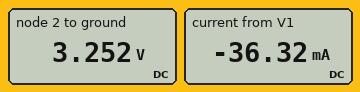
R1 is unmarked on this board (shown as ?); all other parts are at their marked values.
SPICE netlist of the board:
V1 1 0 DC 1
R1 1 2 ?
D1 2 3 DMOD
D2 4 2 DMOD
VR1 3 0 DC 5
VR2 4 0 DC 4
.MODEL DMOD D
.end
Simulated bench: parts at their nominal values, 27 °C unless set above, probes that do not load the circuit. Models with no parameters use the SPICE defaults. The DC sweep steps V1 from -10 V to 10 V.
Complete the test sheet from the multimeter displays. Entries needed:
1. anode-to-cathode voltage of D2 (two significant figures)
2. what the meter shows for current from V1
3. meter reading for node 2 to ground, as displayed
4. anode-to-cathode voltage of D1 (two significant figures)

750 mV
-36.32 mA
3.252 V
-1.7 V
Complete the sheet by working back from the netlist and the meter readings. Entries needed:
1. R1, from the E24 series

62 Ω
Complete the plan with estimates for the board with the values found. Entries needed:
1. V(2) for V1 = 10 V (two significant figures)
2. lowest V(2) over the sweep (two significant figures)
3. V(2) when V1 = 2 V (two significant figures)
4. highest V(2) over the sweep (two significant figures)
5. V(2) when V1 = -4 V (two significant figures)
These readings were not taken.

5.8 V
3.2 V
3.3 V
5.8 V
3.2 V
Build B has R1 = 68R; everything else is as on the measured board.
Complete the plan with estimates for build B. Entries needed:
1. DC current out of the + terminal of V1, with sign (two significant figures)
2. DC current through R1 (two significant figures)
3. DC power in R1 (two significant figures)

-33 mA
33 mA
75 mW
